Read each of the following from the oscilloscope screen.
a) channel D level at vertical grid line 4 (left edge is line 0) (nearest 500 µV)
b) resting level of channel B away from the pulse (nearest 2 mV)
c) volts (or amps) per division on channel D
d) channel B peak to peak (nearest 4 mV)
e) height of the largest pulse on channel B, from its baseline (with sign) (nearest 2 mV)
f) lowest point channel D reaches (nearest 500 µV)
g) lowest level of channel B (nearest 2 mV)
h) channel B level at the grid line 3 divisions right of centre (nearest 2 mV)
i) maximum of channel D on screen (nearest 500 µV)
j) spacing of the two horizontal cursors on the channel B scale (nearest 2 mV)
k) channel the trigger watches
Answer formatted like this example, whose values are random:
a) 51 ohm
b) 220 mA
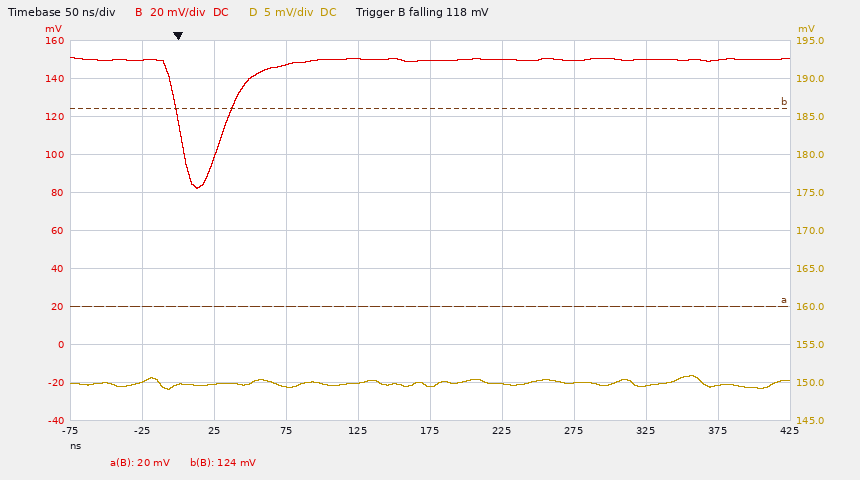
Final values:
a) 150.0 mV
b) 150 mV
c) 5 mV
d) 68 mV
e) -68 mV
f) 149.0 mV
g) 82 mV
h) 150 mV
i) 151.0 mV
j) 104 mV
k) channel B
